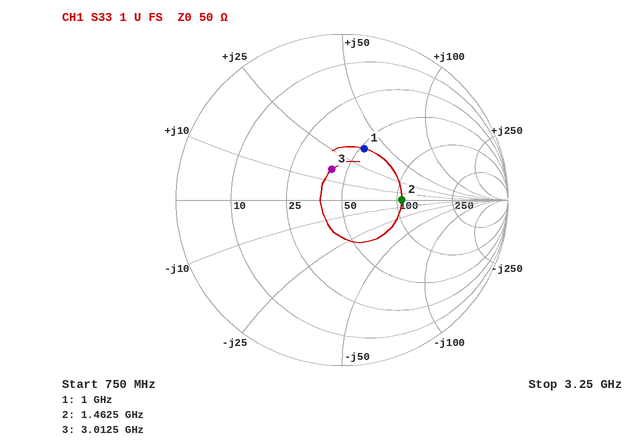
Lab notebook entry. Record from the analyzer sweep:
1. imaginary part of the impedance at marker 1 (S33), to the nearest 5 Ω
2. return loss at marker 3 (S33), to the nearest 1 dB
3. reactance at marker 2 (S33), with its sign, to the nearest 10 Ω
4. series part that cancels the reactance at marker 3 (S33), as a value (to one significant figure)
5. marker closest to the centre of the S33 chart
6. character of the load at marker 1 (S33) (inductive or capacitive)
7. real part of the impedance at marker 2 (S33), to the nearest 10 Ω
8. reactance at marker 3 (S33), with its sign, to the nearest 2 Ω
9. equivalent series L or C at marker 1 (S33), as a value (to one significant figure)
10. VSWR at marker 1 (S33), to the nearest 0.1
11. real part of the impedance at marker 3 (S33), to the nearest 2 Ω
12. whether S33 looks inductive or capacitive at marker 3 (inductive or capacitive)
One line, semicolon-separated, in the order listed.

+35 Ω; 14 dB; 0 Ω; 3 pF; marker 3; inductive; 110 Ω; +16 Ω; 6 nH; 2.0; 42 Ω; inductive
